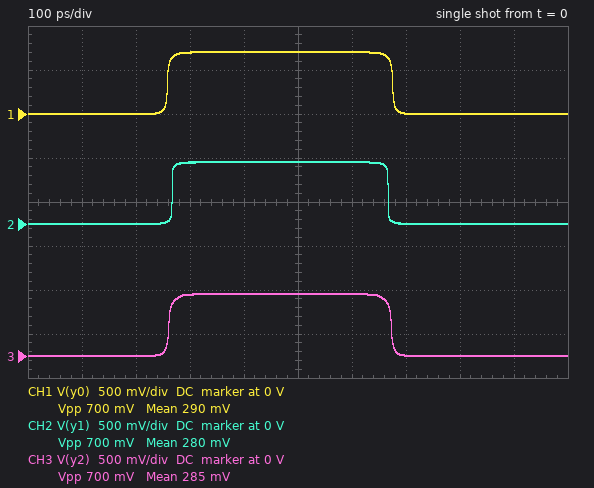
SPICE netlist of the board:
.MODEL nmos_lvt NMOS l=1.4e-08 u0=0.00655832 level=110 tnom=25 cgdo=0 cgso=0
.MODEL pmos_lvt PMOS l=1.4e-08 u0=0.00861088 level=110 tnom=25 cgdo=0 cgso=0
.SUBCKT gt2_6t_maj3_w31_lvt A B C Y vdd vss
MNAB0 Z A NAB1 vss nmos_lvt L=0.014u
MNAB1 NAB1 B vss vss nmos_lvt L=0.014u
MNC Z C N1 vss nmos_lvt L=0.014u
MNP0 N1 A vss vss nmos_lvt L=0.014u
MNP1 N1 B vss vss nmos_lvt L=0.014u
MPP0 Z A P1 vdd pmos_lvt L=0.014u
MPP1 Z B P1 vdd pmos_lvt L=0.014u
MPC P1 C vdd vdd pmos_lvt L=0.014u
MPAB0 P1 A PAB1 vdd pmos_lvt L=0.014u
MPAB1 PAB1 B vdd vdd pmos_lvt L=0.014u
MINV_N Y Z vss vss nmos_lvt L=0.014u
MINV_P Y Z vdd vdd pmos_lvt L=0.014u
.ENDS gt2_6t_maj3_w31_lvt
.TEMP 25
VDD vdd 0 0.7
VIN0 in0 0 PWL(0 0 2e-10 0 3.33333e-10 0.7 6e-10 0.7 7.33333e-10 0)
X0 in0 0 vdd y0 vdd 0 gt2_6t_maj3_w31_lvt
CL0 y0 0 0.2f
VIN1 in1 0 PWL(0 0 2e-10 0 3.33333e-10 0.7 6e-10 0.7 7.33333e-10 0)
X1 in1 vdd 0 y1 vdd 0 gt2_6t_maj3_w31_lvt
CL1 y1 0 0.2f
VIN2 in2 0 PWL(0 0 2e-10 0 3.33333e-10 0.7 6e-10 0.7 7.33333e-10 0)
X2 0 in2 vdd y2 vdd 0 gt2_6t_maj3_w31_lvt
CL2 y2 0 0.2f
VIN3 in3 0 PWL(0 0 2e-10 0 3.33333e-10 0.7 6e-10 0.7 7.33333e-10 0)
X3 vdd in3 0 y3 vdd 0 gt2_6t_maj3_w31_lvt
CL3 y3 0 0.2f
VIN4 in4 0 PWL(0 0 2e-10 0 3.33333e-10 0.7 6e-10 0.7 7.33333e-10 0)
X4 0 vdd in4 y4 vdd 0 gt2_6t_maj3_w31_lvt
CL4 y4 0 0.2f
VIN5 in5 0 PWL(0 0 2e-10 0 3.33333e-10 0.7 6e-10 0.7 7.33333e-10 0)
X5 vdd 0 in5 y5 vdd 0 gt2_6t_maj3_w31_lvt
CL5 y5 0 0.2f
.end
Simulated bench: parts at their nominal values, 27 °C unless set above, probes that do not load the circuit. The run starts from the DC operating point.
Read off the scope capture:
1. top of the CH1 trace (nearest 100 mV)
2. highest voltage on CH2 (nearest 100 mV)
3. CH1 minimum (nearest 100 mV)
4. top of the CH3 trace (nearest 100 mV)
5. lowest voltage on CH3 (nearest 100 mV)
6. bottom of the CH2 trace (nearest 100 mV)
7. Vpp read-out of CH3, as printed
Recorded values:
700 mV
700 mV
0 V
700 mV
0 V
0 V
700 mV
